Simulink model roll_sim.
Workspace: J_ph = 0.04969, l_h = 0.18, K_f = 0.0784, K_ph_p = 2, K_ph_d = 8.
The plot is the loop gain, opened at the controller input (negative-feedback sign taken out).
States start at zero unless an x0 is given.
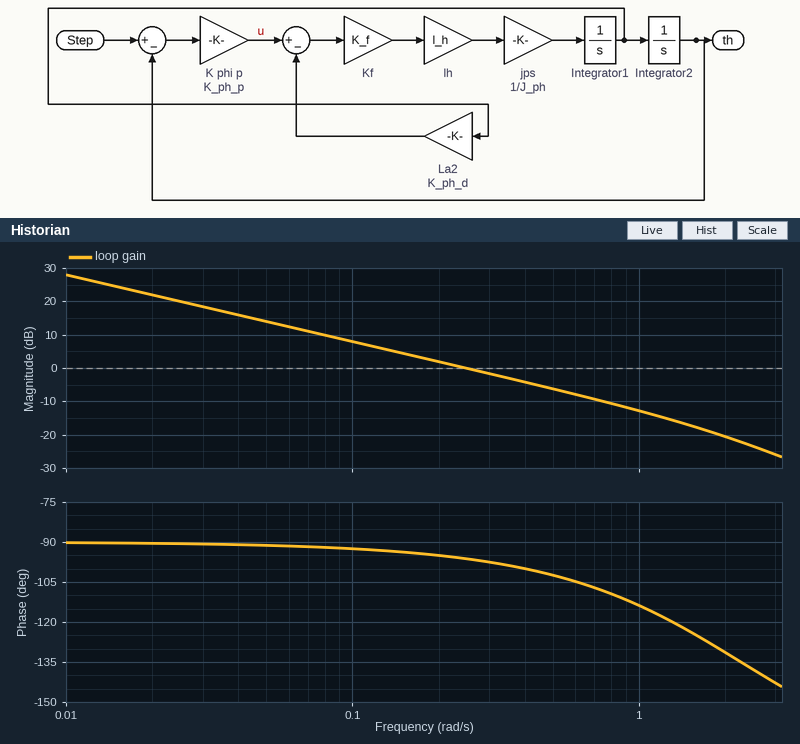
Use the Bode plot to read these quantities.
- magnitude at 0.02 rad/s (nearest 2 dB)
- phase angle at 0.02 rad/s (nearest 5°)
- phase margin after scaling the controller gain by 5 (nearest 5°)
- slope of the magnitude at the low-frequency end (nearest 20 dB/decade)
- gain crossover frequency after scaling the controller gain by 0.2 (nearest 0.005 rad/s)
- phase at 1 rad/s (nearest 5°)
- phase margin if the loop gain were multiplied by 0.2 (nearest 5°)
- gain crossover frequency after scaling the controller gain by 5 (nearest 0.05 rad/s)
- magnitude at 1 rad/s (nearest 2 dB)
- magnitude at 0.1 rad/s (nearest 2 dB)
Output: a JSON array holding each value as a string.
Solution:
["22 dB", "-90°", "65°", "-20 dB/decade", "0.050 rad/s", "-115°", "90°", "1.10 rad/s", "-12 dB", "8 dB"]
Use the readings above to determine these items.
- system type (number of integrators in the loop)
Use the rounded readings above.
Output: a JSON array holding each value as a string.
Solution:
["1"]
